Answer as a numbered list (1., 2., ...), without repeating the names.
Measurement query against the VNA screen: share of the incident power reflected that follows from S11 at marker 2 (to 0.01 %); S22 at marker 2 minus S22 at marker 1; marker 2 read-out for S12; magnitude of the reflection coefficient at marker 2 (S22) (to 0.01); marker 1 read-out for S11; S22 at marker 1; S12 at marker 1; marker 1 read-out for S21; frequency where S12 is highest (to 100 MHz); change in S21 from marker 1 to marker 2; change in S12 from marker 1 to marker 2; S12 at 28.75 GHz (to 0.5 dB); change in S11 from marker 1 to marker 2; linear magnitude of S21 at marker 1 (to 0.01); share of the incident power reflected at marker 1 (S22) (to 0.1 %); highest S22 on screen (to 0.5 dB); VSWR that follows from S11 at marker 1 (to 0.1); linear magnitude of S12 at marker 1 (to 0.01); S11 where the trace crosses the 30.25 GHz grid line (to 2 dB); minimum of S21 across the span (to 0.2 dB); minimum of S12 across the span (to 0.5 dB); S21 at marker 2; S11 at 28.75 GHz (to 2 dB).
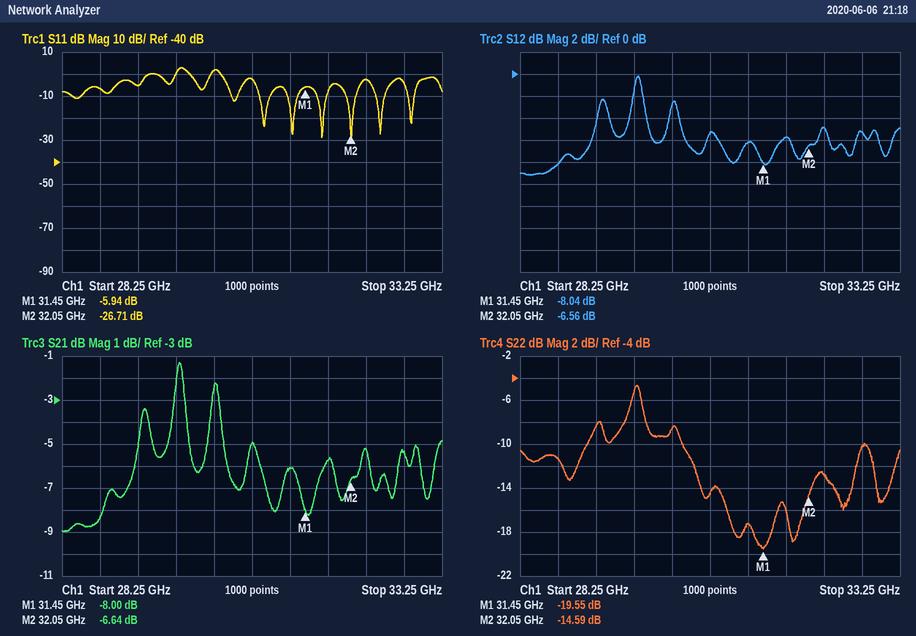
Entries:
1. 0.21 %
2. 4.96 dB
3. -6.56 dB
4. 0.19
5. -5.94 dB
6. -19.55 dB
7. -8.04 dB
8. -8.00 dB
9. 29.8 GHz
10. 1.36 dB
11. 1.48 dB
12. -8.0 dB
13. -20.77 dB
14. 0.40
15. 1.1 %
16. -4.5 dB
17. 3.0
18. 0.40
19. 2 dB
20. -9.0 dB
21. -9.0 dB
22. -6.64 dB
23. -6 dB
